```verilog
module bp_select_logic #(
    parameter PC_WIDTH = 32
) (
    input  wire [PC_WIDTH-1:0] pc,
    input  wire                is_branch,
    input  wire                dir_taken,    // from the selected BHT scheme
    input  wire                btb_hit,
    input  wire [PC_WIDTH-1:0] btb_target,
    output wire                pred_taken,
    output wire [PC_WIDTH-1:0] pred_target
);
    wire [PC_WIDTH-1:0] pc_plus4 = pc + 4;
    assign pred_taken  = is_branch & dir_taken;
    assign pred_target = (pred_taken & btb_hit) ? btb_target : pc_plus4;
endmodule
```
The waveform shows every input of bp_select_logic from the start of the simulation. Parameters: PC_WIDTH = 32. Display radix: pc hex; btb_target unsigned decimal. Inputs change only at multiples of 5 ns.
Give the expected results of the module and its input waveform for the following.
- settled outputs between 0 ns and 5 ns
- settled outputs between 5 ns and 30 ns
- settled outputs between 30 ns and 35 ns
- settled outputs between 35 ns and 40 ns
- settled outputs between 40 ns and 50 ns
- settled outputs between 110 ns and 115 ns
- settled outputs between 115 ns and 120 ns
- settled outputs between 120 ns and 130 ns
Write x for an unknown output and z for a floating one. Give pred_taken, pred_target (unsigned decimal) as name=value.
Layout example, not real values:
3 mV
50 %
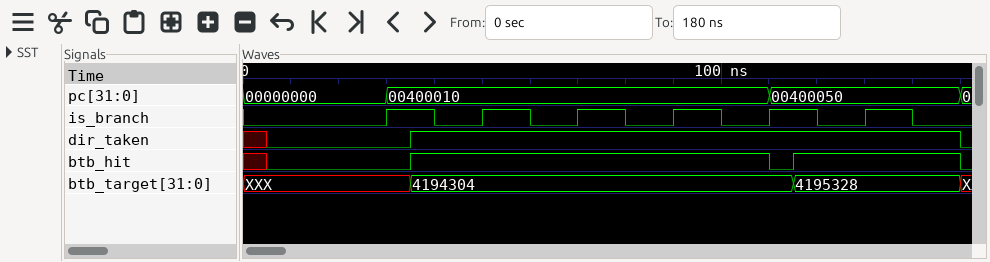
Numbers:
pred_taken=0, pred_target=4
pred_taken=0, pred_target=4
pred_taken=0, pred_target=4194324
pred_taken=1, pred_target=4194304
pred_taken=0, pred_target=4194324
pred_taken=1, pred_target=4194388
pred_taken=1, pred_target=4195328
pred_taken=0, pred_target=4194388
